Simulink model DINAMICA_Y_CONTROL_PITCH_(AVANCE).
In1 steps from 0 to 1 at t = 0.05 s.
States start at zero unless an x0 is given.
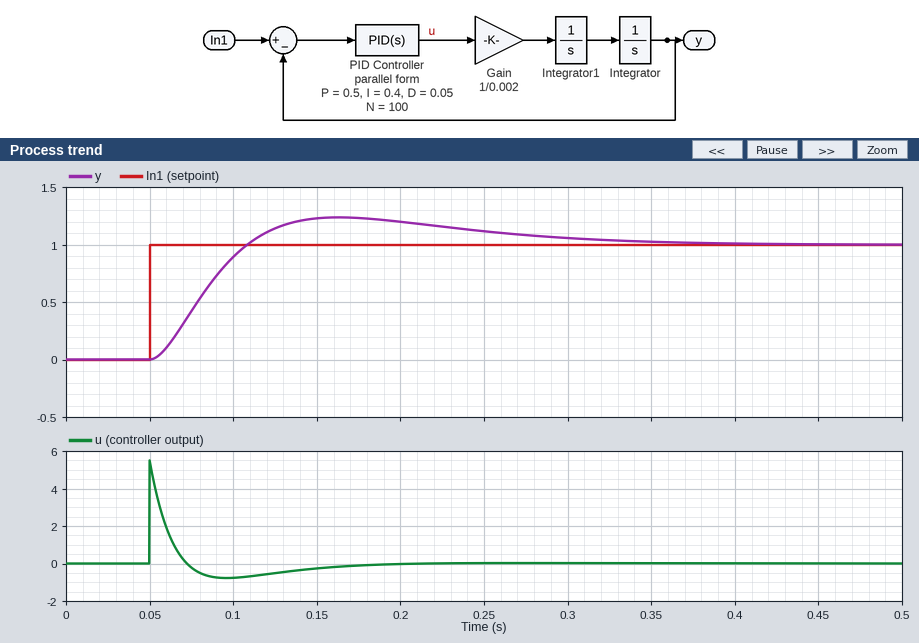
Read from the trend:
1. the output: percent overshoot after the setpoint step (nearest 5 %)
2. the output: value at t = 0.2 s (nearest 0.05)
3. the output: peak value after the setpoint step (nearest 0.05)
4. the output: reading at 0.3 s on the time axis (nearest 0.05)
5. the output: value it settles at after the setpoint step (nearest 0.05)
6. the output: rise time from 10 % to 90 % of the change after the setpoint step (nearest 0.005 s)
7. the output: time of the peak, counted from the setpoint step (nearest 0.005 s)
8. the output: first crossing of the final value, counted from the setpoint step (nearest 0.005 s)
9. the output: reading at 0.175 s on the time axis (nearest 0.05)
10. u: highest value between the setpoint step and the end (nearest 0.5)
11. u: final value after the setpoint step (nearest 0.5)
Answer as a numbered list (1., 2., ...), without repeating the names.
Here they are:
1. 25 %
2. 1.20
3. 1.25
4. 1.05
5. 1.00
6. 0.040 s
7. 0.115 s
8. 0.060 s
9. 1.25
10. 5.5
11. 0.0
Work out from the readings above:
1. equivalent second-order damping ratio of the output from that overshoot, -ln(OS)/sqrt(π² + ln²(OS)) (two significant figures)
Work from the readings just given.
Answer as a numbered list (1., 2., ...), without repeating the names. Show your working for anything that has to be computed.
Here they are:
1. ln(0.25) = -1.386; 1.386 / sqrt(9.870 + 1.922) = 0.40
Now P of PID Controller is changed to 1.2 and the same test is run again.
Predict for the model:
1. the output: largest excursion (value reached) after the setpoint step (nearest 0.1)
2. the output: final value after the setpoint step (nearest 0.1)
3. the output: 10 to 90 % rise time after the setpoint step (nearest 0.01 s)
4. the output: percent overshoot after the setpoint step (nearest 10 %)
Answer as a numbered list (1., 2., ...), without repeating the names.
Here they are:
1. 1.4
2. 1.0
3. 0.03 s
4. 40 %
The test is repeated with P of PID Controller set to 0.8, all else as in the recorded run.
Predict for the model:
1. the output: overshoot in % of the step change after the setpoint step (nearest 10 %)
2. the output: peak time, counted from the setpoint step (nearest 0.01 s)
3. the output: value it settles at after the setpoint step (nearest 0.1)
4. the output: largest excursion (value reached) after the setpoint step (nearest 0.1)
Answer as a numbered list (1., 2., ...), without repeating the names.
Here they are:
1. 30 %
2. 0.10 s
3. 1.0
4. 1.3
